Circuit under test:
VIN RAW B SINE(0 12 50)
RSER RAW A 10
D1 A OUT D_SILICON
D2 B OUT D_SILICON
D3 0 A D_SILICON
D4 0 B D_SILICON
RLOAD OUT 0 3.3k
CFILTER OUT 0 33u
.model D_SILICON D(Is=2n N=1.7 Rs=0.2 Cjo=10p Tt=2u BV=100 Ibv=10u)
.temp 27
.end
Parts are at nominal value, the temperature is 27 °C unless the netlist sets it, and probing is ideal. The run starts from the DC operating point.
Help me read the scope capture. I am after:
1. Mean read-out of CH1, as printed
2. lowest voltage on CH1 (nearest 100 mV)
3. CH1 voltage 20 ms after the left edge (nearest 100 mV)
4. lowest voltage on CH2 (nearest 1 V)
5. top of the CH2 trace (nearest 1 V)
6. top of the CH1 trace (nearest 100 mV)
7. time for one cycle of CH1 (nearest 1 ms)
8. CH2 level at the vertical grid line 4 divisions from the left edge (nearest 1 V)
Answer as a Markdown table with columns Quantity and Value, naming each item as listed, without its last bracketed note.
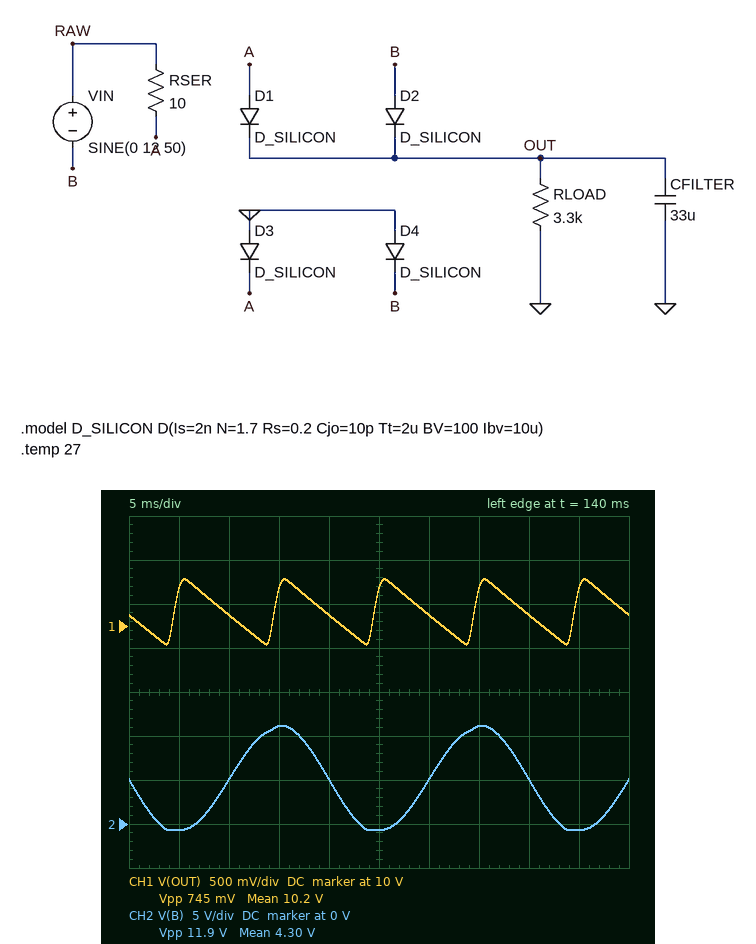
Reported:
| Quantity | Value |
|---|---|
| Mean read-out of CH1, as printed | 10.2 V |
| lowest voltage on CH1 | 9.8 V |
| CH1 voltage 20 ms after the left edge | 10.1 V |
| lowest voltage on CH2 | -1 V |
| top of the CH2 trace | 11 V |
| top of the CH1 trace | 10.5 V |
| time for one cycle of CH1 | 10 ms |
| CH2 level at the vertical grid line 4 divisions from the left edge | 5 V |
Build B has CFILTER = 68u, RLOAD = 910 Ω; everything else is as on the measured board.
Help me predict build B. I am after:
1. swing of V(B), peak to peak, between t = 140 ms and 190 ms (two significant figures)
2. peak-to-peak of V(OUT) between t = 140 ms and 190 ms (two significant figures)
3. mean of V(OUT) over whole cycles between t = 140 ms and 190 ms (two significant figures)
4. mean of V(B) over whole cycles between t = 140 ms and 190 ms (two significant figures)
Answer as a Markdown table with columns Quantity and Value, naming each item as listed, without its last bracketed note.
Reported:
| Quantity | Value |
|---|---|
| swing of V(B), peak to peak, between t = 140 ms and 190 ms | 12 V |
| peak-to-peak of V(OUT) between t = 140 ms and 190 ms | 1.2 V |
| mean of V(OUT) over whole cycles between t = 140 ms and 190 ms | 9.6 V |
| mean of V(B) over whole cycles between t = 140 ms and 190 ms | 4.8 V |
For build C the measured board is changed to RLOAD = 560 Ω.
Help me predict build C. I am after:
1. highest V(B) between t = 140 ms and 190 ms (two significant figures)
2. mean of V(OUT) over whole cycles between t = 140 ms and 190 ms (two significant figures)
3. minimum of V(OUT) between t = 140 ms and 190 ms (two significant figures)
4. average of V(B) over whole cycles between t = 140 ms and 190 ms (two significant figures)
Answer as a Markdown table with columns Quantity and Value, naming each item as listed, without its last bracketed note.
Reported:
| Quantity | Value |
|---|---|
| highest V(B) between t = 140 ms and 190 ms | 11 V |
| mean of V(OUT) over whole cycles between t = 140 ms and 190 ms | 8.8 V |
| minimum of V(OUT) between t = 140 ms and 190 ms | 7.1 V |
| average of V(B) over whole cycles between t = 140 ms and 190 ms | 4.4 V |
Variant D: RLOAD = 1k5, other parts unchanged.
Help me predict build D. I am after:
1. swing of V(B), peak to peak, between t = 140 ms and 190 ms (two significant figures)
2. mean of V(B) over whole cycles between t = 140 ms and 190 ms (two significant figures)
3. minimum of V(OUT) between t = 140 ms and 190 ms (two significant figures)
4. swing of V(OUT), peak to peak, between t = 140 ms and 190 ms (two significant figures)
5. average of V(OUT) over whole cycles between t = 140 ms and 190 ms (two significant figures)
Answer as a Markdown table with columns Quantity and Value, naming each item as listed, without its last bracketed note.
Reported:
| Quantity | Value |
|---|---|
| swing of V(B), peak to peak, between t = 140 ms and 190 ms | 12 V |
| mean of V(B) over whole cycles between t = 140 ms and 190 ms | 4.9 V |
| minimum of V(OUT) between t = 140 ms and 190 ms | 9.0 V |
| swing of V(OUT), peak to peak, between t = 140 ms and 190 ms | 1.5 V |
| average of V(OUT) over whole cycles between t = 140 ms and 190 ms | 9.7 V |
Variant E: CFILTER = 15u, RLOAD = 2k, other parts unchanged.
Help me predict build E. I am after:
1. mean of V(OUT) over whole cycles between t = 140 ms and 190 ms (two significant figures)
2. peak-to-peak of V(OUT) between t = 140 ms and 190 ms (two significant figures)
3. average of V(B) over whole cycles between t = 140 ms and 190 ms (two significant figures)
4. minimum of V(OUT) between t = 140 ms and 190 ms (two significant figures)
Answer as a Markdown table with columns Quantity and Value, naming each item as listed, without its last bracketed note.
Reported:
| Quantity | Value |
|---|---|
| mean of V(OUT) over whole cycles between t = 140 ms and 190 ms | 9.5 V |
| peak-to-peak of V(OUT) between t = 140 ms and 190 ms | 2.3 V |
| average of V(B) over whole cycles between t = 140 ms and 190 ms | 4.7 V |
| minimum of V(OUT) between t = 140 ms and 190 ms | 8.3 V |
